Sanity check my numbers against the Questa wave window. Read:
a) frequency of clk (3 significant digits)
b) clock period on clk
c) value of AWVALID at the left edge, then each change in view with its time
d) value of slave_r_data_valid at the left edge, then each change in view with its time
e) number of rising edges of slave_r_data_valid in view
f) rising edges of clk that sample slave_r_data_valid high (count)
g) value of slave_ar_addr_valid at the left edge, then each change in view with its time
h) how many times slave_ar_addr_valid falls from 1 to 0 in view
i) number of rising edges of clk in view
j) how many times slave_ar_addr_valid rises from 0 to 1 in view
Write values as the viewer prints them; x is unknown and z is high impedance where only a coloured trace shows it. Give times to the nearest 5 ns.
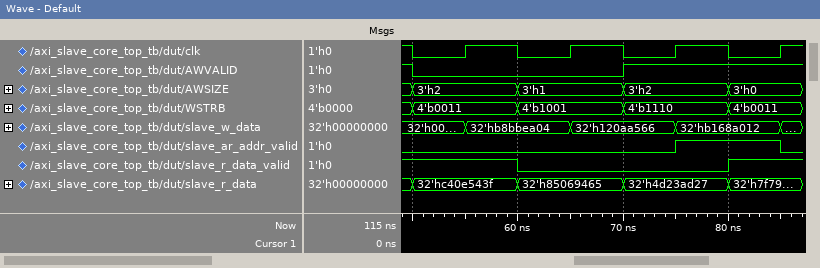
100 MHz
10 ns
1, 0 at 50 ns, 1 at 70 ns
1, 0 at 60 ns, 1 at 80 ns
1
2
0, 1 at 75 ns, 0 at 85 ns
1
4
1
